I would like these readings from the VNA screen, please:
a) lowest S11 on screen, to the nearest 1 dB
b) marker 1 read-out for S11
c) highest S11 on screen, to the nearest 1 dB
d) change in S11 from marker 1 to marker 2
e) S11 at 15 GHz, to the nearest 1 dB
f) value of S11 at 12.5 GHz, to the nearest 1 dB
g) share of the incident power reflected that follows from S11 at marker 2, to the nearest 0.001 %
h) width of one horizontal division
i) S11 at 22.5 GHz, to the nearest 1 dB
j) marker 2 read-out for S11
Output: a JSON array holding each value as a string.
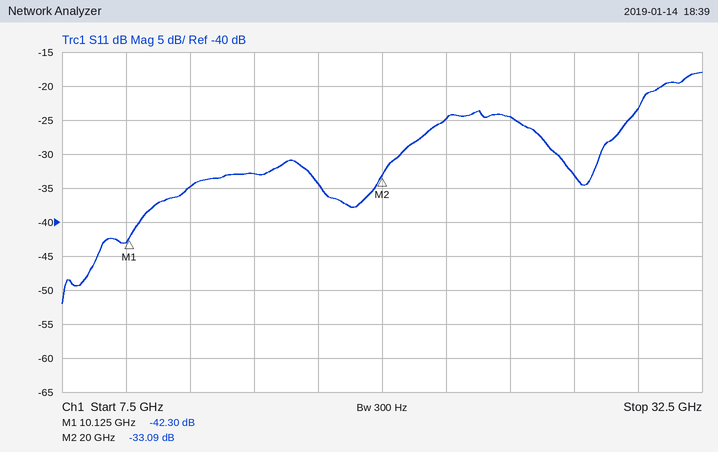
["-52 dB", "-42.30 dB", "-18 dB", "9.21 dB", "-33 dB", "-35 dB", "0.049 %", "2.5 GHz", "-25 dB", "-33.09 dB"]
